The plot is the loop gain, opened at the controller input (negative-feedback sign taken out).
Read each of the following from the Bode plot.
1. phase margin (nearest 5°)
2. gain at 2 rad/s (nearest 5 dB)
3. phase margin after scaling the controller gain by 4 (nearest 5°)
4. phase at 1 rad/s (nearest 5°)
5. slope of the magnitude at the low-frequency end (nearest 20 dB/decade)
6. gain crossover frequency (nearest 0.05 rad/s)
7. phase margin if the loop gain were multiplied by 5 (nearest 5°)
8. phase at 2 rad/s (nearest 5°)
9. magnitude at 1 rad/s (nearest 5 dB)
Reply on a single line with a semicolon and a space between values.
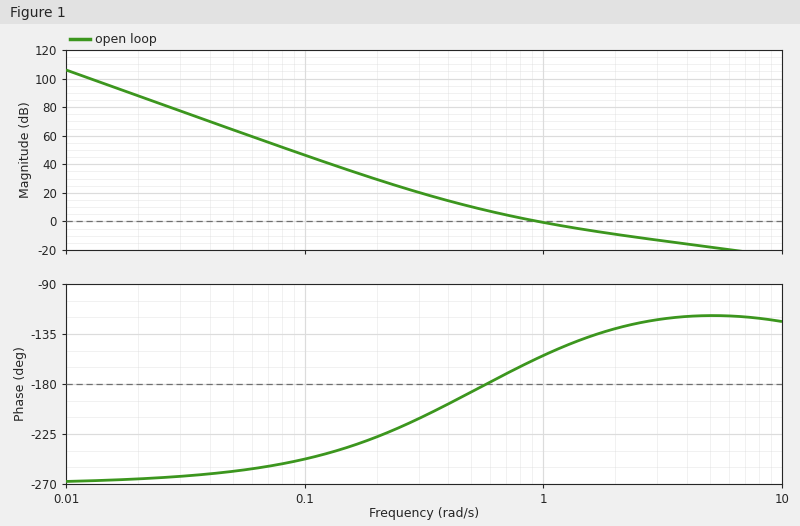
25°; -10 dB; 55°; -155°; -60 dB/decade; 0.95 rad/s; 60°; -130°; 0 dB
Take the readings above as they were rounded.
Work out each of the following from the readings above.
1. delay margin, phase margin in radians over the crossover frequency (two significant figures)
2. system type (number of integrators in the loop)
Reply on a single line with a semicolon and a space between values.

0.46 s; 3
